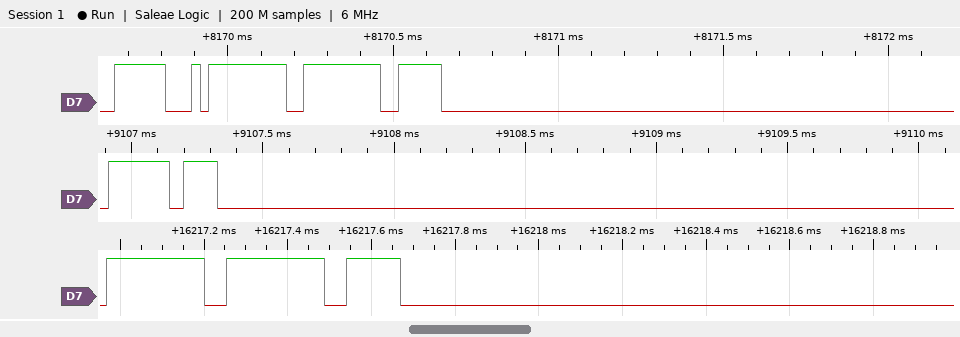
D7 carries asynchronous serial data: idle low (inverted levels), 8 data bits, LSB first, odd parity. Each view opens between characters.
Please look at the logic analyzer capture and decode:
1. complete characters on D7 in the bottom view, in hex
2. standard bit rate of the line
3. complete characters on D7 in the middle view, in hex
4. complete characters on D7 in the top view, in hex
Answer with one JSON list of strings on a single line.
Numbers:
["00, 00, F0", "38400 baud", "00, F0", "E0, 00, 00, F0"]
